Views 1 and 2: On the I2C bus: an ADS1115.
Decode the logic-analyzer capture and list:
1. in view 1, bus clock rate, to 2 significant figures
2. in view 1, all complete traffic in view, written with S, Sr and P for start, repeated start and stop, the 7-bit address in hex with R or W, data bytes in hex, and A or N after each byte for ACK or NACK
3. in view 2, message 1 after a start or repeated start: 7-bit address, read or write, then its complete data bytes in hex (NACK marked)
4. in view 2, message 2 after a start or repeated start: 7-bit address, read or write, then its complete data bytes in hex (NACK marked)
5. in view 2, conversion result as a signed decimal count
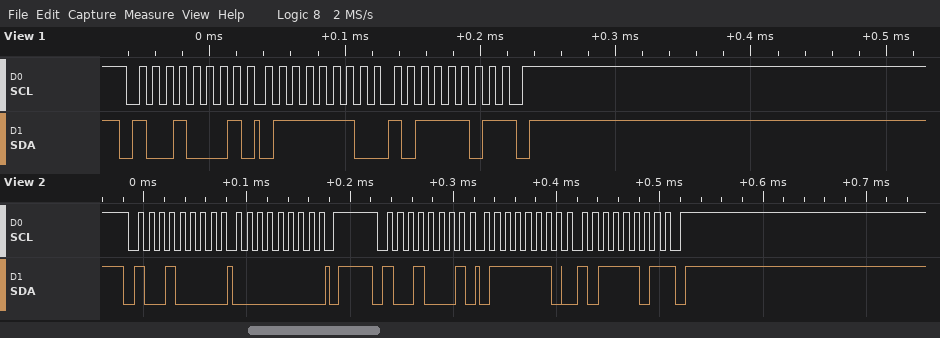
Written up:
100 kHz
S 48R A 7E A BD N P
0x48 write: 00
0x48 read: 7E BD NACK
32445
